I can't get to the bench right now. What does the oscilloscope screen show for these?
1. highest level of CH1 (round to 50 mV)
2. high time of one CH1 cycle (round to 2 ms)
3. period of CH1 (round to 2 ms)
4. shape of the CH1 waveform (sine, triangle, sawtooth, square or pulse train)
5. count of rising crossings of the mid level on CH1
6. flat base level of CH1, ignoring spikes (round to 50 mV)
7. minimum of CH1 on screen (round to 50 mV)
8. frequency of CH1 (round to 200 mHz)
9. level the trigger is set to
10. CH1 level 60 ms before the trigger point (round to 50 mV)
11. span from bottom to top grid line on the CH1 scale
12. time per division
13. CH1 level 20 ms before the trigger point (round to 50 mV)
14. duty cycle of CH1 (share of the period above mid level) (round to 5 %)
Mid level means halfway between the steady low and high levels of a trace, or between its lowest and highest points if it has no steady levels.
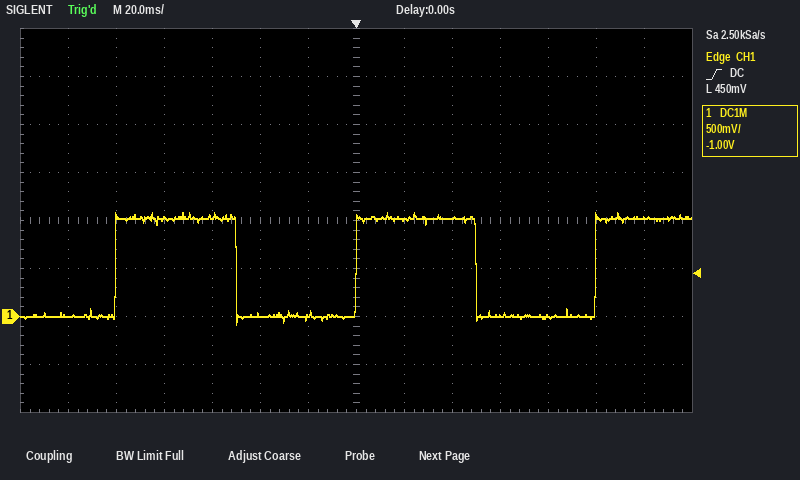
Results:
1.10 V
50 ms
100 ms
square
3
0 mV
-100 mV
10.0 Hz
450 mV
1.05 V
4 V
20 ms
0 mV
50 %
